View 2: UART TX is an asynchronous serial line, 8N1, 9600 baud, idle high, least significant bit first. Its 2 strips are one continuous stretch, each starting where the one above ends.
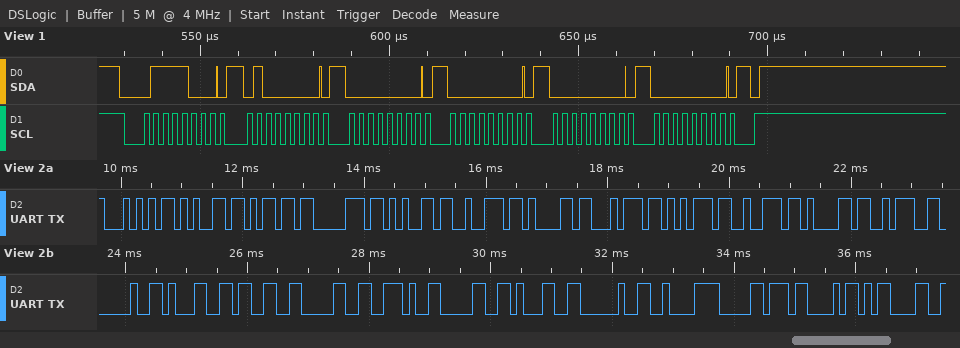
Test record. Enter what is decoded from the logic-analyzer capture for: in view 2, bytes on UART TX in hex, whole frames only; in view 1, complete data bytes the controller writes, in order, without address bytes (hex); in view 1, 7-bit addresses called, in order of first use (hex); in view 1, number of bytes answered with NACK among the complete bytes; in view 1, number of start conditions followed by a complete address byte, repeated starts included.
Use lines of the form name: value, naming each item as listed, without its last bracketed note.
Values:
in view 2, bytes on UART TX in hex, whole frames only: 0x54 0x65 0x6D 0x70 0x65 0x72 0x61 0x74 0x75 0x72 0x61 0x3A 0x20 0x31 0x33 0x30 0x2E 0x30 0x31 0x20 0xC2 0xB0 0x43 0x0D
in view 1, complete data bytes the controller writes, in order, without address bytes: 40 00 00 00 00
in view 1, 7-bit addresses called, in order of first use: 0x3C
in view 1, number of bytes answered with NACK among the complete bytes: 0
in view 1, number of start conditions followed by a complete address byte, repeated starts included: 1
